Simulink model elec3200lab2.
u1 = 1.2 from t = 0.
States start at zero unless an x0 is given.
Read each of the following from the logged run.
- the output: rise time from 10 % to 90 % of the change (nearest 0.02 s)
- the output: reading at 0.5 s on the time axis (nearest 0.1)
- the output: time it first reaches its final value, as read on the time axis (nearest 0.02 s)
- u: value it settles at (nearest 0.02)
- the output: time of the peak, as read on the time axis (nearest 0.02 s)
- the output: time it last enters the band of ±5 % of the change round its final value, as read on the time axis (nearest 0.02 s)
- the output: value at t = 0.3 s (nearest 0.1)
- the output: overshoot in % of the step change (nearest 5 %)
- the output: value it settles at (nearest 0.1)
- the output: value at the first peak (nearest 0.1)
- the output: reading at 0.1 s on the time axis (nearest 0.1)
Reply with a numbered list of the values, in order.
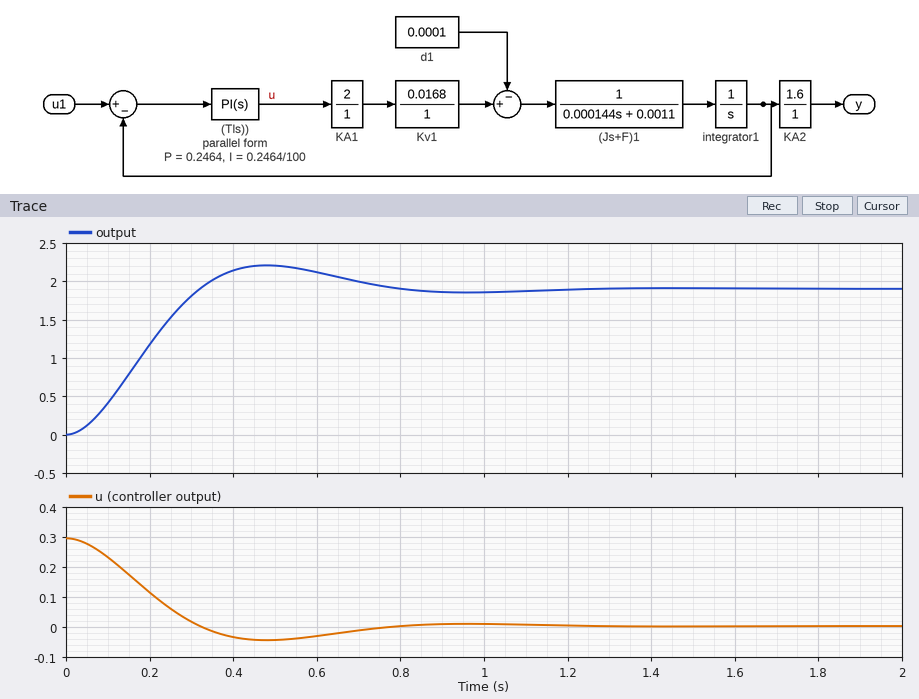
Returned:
1. 0.22 s
2. 2.2
3. 0.32 s
4. 0.00
5. 0.48 s
6. 0.70 s
7. 1.8
8. 15 %
9. 1.9
10. 2.2
11. 0.4
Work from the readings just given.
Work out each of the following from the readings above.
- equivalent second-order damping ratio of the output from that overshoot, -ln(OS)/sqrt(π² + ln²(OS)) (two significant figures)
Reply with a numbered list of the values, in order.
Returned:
1. 0.52
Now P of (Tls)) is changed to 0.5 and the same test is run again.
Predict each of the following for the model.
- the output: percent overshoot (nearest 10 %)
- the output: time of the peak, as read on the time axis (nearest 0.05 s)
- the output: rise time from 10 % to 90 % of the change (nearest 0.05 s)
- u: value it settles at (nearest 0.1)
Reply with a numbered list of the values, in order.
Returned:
1. 30 %
2. 0.30 s
3. 0.15 s
4. 0.0
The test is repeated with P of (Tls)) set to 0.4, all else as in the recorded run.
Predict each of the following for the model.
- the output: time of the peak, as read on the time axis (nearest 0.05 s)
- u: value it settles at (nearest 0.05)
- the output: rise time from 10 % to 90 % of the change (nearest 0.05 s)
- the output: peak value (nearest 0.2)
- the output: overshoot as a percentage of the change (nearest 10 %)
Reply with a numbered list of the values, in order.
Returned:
1. 0.35 s
2. 0.00
3. 0.15 s
4. 2.4
5. 30 %
